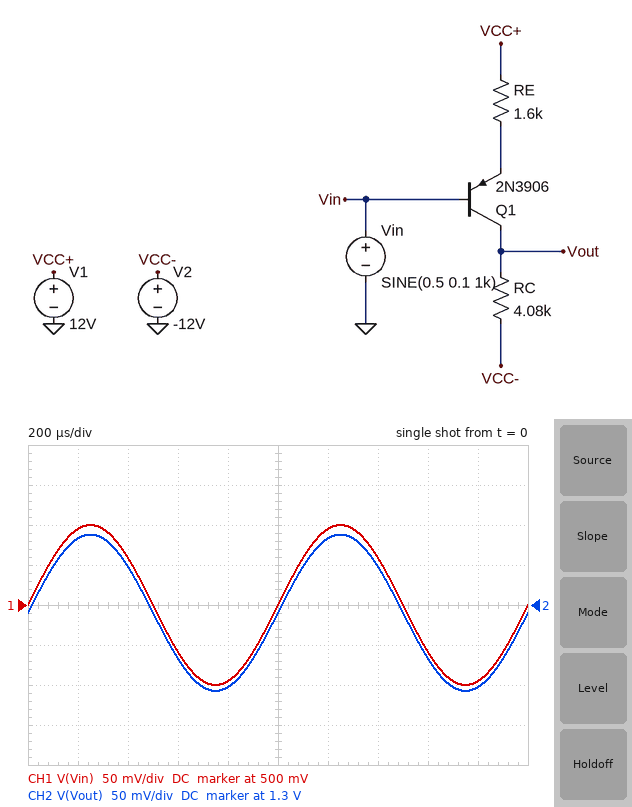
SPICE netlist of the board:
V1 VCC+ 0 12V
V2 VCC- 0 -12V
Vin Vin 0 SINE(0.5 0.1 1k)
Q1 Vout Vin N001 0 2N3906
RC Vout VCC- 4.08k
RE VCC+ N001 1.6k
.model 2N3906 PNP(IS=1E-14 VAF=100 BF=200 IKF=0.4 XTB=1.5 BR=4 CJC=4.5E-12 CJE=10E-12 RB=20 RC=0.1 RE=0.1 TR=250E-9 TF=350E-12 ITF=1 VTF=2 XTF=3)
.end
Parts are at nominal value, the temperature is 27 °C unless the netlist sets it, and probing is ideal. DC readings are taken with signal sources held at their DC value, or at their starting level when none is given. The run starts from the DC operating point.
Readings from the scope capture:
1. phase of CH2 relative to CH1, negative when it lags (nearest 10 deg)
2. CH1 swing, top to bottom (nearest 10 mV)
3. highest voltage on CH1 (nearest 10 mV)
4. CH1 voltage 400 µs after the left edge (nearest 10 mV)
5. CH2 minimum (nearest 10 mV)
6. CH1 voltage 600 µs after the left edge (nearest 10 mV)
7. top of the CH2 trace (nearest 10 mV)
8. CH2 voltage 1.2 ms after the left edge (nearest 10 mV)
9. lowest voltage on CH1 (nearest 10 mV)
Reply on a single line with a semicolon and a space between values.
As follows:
0 deg; 200 mV; 600 mV; 560 mV; 1.19 V; 440 mV; 1.39 V; 1.38 V; 400 mV
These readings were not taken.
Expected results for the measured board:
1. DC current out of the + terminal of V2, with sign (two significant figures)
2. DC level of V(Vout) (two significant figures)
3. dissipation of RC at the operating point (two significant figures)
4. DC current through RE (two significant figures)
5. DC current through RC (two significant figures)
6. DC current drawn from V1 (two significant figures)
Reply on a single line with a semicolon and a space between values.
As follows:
-3.3 mA; 1.3 V; 43 mW; 6.7 mA; 3.3 mA; 6.7 mA
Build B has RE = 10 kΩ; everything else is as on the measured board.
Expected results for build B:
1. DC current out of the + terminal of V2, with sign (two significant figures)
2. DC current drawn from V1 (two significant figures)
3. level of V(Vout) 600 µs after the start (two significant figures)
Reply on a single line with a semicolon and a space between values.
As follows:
-1.1 mA; 1.1 mA; -7.6 V
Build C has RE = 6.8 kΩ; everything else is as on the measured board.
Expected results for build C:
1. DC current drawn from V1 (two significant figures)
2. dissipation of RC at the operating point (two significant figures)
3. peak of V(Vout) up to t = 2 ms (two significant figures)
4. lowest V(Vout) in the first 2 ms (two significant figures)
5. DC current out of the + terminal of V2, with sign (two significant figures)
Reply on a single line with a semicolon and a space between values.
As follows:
1.6 mA; 10 mW; -5.5 V; -5.6 V; -1.6 mA
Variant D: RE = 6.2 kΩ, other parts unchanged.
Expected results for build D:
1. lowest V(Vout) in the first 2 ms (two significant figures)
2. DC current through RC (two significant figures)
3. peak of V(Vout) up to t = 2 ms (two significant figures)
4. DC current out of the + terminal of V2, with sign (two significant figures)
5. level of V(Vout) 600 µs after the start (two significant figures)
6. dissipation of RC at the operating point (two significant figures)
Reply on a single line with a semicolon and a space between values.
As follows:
-5.0 V; 1.7 mA; -4.8 V; -1.7 mA; -4.9 V; 12 mW
